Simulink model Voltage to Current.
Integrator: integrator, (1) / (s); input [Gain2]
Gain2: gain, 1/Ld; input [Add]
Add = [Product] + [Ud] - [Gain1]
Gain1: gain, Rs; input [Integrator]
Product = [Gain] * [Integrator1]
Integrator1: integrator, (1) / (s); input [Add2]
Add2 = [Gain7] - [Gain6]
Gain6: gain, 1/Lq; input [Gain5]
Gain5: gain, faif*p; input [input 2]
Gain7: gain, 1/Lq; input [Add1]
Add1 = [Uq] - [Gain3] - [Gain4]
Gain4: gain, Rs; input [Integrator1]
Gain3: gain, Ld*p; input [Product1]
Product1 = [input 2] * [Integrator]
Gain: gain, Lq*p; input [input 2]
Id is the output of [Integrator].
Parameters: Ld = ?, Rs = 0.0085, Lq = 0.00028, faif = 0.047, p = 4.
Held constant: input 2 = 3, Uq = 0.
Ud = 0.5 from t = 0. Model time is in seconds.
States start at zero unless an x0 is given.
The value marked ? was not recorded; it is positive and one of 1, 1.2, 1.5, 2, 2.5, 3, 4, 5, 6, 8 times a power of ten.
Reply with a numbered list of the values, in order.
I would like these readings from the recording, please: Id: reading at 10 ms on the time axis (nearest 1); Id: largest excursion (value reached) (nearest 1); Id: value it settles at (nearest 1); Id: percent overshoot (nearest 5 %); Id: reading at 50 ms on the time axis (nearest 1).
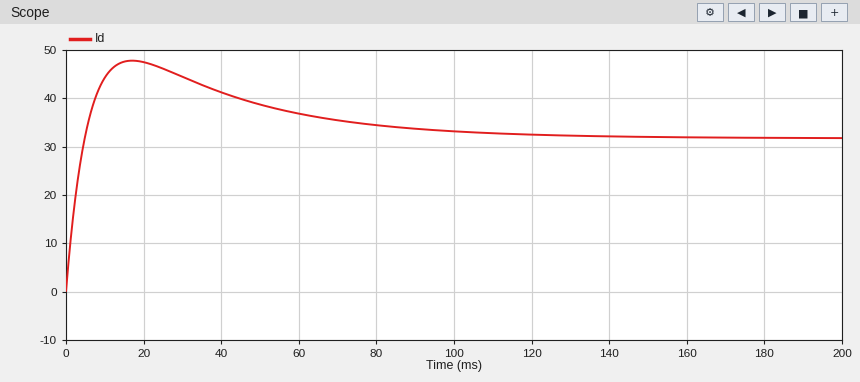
1. 44
2. 48
3. 32
4. 50 %
5. 39
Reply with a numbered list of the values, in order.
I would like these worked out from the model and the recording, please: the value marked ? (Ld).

1. 5e-05
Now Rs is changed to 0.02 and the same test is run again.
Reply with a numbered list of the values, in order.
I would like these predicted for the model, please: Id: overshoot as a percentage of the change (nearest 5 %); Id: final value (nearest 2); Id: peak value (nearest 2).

1. 10 %
2. 20
3. 22
